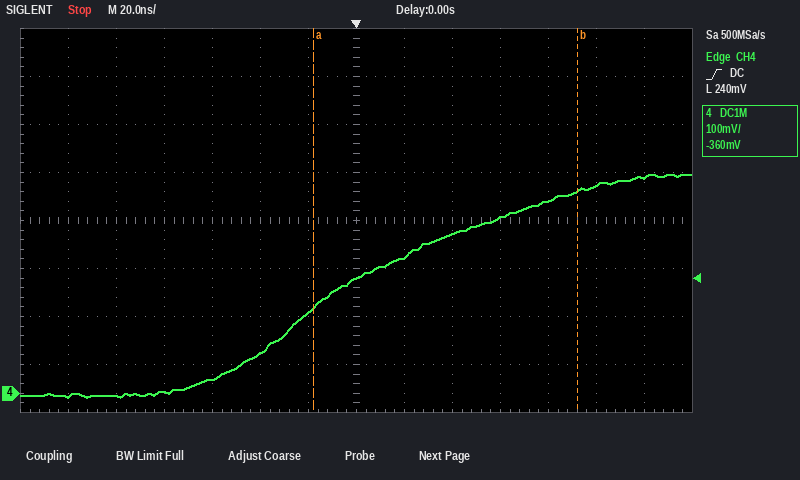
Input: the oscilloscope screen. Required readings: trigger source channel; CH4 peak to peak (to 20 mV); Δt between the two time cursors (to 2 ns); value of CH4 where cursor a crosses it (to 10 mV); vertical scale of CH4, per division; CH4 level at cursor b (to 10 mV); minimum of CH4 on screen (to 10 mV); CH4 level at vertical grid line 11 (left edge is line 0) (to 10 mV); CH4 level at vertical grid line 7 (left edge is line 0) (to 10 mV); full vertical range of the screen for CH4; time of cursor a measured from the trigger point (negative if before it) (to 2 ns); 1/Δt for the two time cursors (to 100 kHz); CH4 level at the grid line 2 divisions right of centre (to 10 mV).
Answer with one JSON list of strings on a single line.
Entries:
["CH4", "460 mV", "110 ns", "180 mV", "100 mV", "420 mV", "-10 mV", "400 mV", "240 mV", "800 mV", "-18 ns", "9.1 MHz", "330 mV"]
